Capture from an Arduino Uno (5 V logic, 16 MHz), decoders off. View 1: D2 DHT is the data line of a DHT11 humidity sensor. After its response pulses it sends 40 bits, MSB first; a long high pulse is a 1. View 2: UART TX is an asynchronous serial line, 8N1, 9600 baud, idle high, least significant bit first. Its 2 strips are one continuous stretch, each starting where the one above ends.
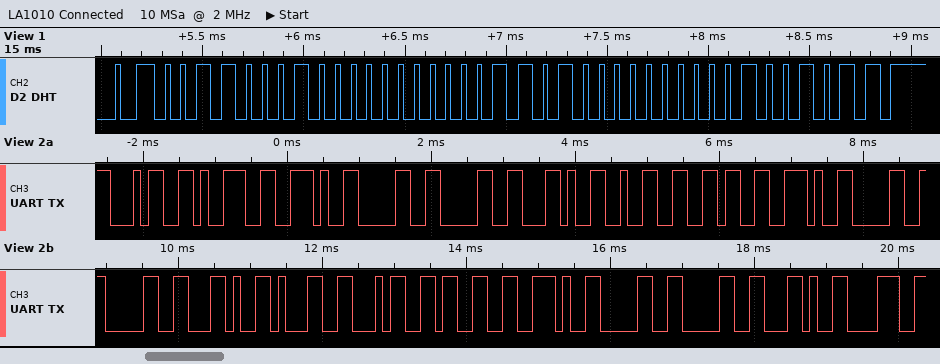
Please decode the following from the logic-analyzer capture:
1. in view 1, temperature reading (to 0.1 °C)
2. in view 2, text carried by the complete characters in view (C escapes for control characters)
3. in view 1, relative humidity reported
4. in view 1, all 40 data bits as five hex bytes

26.0 °C
"49.00,26.00,143.00,8"
49 %
31 00 1A 00 4B
